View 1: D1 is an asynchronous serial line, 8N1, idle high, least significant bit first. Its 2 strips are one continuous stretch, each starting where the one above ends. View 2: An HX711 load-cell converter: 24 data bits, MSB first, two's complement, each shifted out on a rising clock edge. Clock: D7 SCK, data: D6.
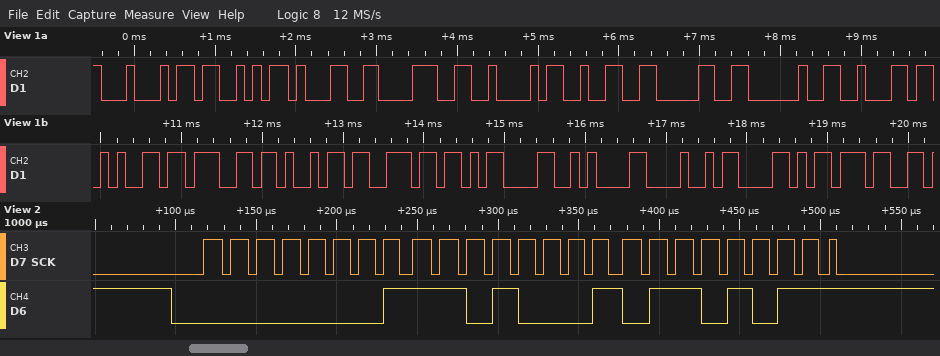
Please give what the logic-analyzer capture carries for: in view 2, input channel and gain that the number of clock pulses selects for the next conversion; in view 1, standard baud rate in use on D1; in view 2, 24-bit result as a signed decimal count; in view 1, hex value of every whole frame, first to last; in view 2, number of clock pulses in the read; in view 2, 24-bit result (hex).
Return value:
channel A, gain 128
9600 baud
119147
44 53 31 38 42 32 30 20 62 65 67 69 6E 0D 0A 48 58 37
25
0x01D16B
